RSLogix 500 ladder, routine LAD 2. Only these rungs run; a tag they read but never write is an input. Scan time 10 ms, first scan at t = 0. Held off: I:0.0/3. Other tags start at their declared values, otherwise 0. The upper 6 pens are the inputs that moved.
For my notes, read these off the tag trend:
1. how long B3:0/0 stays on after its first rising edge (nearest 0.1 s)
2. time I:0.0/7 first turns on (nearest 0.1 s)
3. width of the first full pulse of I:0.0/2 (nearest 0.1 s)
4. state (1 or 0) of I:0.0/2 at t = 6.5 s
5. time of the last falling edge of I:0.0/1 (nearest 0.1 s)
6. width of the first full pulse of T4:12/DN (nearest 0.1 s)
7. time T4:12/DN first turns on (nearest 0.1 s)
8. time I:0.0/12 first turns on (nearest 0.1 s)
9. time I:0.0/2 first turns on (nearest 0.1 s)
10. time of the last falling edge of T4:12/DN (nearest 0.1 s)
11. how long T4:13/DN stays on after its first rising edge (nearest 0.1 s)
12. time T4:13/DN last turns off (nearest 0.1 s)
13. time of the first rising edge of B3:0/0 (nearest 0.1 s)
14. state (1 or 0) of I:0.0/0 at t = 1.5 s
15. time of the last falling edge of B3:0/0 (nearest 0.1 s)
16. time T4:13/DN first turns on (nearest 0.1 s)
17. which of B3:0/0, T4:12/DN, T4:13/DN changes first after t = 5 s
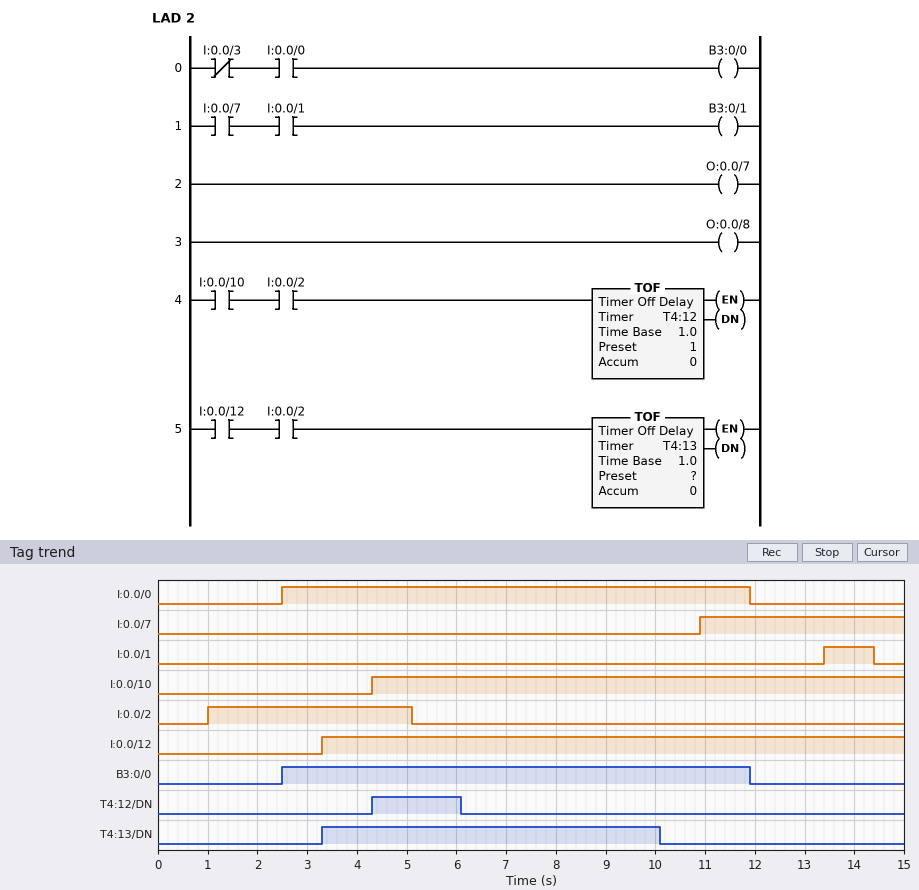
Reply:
9.4 s
10.9 s
4.1 s
0
14.4 s
1.8 s
4.3 s
3.3 s
1.0 s
6.1 s
6.8 s
10.1 s
2.5 s
0
11.9 s
3.3 s
T4:12/DN
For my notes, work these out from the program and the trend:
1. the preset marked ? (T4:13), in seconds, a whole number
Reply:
5 s
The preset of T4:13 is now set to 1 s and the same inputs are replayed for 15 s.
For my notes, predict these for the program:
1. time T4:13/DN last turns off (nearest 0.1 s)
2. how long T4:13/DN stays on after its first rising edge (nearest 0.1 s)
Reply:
6.1 s
2.8 s
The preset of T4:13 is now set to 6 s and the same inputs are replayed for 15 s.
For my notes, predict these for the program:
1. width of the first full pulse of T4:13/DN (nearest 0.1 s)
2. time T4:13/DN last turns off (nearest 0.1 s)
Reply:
7.8 s
11.1 s
